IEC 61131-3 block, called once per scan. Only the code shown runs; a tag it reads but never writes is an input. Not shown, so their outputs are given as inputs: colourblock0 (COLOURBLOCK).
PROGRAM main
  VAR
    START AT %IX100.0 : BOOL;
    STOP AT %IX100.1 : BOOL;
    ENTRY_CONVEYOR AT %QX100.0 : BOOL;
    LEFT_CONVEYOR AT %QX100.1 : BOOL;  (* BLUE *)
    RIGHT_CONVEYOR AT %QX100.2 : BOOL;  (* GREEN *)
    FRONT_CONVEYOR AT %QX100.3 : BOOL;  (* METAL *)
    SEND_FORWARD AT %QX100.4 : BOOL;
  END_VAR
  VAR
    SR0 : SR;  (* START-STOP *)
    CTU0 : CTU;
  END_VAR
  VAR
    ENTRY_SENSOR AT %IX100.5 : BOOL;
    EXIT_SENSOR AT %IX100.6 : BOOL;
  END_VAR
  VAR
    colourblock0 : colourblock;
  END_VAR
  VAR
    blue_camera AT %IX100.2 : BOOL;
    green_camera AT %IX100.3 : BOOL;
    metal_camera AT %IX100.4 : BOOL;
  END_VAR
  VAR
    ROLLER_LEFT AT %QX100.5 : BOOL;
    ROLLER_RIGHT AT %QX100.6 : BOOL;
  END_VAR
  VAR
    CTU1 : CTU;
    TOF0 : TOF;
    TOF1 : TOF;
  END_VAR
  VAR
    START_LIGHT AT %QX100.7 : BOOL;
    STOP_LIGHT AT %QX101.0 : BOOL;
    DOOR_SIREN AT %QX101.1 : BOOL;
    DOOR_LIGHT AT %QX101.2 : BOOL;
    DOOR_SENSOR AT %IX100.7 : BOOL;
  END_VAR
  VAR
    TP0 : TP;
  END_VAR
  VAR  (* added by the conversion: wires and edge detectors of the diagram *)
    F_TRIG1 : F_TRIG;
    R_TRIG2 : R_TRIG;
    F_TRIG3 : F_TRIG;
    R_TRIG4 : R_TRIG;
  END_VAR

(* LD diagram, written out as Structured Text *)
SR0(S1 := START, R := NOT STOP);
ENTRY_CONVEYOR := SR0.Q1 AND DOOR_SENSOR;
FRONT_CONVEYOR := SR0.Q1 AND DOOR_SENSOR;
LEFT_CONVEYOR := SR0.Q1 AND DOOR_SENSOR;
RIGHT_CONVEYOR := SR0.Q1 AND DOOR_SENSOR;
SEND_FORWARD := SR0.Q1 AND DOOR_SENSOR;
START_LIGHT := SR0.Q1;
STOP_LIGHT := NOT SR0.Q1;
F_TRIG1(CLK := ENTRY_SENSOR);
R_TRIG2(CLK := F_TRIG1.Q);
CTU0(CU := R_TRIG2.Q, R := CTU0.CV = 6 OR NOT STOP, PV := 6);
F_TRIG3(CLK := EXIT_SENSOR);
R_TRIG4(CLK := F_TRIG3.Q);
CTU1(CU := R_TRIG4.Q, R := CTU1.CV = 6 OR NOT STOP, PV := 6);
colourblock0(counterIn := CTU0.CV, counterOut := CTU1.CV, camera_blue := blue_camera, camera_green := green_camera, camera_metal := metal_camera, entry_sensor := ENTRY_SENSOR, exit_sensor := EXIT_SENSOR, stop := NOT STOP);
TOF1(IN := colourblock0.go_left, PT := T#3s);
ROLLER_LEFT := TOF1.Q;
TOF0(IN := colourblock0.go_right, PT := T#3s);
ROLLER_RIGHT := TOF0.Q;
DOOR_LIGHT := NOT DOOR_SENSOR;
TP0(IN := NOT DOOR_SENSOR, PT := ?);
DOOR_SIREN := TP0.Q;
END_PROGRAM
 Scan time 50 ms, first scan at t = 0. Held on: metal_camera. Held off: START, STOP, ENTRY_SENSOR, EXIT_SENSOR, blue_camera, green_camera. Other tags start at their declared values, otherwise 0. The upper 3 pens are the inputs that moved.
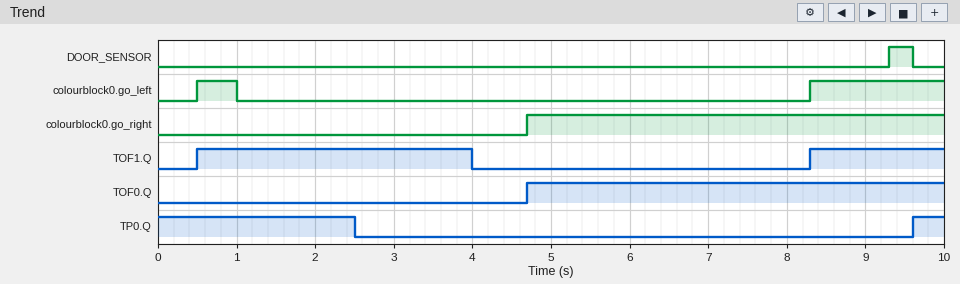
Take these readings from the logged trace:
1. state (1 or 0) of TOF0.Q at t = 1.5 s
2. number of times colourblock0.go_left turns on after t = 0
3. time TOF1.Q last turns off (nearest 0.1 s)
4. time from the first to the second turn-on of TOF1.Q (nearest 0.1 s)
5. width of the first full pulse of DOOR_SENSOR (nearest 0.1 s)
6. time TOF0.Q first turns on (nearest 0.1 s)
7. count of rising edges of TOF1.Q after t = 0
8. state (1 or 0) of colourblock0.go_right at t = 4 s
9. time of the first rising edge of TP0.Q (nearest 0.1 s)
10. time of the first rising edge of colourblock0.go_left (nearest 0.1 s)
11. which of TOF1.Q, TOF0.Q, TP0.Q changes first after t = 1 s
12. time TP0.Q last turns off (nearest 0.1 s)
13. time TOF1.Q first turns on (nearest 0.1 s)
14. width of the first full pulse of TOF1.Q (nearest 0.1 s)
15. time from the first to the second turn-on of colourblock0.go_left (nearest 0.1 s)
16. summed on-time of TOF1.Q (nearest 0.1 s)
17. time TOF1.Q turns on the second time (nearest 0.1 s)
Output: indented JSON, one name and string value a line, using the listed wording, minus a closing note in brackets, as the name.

{
  "state (1 or 0) of TOF0.Q at t = 1.5 s": "0",
  "number of times colourblock0.go_left turns on after t = 0": "2",
  "time TOF1.Q last turns off": "4.0 s",
  "time from the first to the second turn-on of TOF1.Q": "7.8 s",
  "width of the first full pulse of DOOR_SENSOR": "0.3 s",
  "time TOF0.Q first turns on": "4.7 s",
  "count of rising edges of TOF1.Q after t = 0": "2",
  "state (1 or 0) of colourblock0.go_right at t = 4 s": "0",
  "time of the first rising edge of TP0.Q": "9.6 s",
  "time of the first rising edge of colourblock0.go_left": "0.5 s",
  "which of TOF1.Q, TOF0.Q, TP0.Q changes first after t = 1 s": "TP0.Q",
  "time TP0.Q last turns off": "2.5 s",
  "time TOF1.Q first turns on": "0.5 s",
  "width of the first full pulse of TOF1.Q": "3.5 s",
  "time from the first to the second turn-on of colourblock0.go_left": "7.8 s",
  "summed on-time of TOF1.Q": "5.2 s",
  "time TOF1.Q turns on the second time": "8.3 s"
}
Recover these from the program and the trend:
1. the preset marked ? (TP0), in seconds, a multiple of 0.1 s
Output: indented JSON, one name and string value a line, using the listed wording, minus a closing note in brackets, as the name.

{
  "the preset marked ? (TP0), in seconds, a multiple of 0.1 s": "2.5 s"
}
